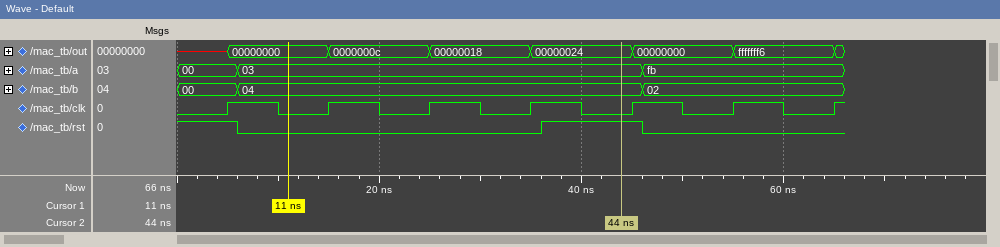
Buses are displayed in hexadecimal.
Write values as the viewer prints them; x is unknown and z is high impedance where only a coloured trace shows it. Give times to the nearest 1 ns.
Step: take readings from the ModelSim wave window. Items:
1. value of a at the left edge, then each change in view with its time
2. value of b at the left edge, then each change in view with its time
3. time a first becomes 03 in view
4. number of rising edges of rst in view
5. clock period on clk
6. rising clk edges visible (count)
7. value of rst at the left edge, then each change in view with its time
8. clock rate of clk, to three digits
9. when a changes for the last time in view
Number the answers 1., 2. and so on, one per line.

1. 00, 03 at 6 ns, fb at 46 ns
2. 00, 04 at 6 ns, 02 at 46 ns
3. 6 ns
4. 1
5. 10 ns
6. 7
7. 1, 0 at 6 ns, 1 at 36 ns, 0 at 46 ns
8. 100 MHz
9. 46 ns
